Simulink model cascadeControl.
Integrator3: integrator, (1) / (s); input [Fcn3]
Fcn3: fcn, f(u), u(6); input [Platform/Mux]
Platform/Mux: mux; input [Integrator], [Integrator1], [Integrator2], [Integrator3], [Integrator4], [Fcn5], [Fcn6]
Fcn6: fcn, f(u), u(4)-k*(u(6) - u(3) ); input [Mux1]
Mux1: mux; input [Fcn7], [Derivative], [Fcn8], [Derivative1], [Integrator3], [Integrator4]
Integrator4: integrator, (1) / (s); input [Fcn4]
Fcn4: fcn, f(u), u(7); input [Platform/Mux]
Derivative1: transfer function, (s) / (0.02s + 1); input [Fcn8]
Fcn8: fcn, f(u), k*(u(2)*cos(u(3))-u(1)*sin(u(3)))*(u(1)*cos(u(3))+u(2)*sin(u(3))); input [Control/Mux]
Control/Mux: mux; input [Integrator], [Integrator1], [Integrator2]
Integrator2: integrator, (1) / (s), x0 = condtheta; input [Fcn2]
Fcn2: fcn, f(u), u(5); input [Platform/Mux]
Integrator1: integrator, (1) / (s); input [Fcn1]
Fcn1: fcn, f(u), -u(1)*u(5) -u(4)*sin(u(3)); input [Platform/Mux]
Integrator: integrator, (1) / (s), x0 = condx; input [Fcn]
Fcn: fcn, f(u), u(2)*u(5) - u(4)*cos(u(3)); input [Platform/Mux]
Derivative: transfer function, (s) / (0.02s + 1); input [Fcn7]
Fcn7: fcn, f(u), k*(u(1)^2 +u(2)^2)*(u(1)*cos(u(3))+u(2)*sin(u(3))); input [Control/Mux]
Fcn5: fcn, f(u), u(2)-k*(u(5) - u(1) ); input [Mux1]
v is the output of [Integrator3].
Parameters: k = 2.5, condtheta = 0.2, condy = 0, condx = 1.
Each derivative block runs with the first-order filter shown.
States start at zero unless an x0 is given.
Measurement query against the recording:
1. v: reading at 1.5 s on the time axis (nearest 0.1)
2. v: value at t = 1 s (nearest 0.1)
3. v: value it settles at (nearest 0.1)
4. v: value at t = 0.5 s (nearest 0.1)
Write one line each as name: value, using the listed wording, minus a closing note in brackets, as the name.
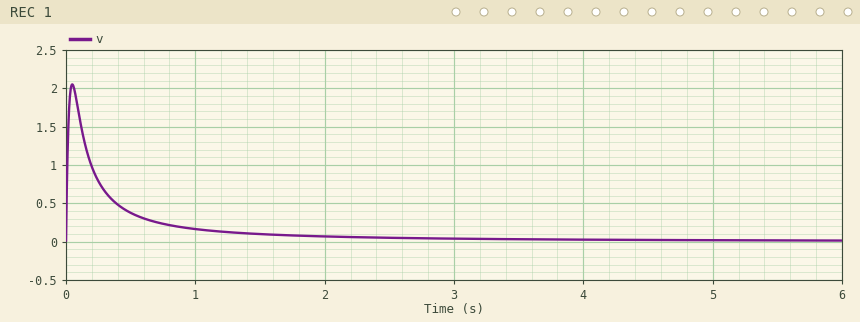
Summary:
v: reading at 1.5 s on the time axis: 0.1
v: value at t = 1 s: 0.2
v: value it settles at: 0.0
v: value at t = 0.5 s: 0.4
